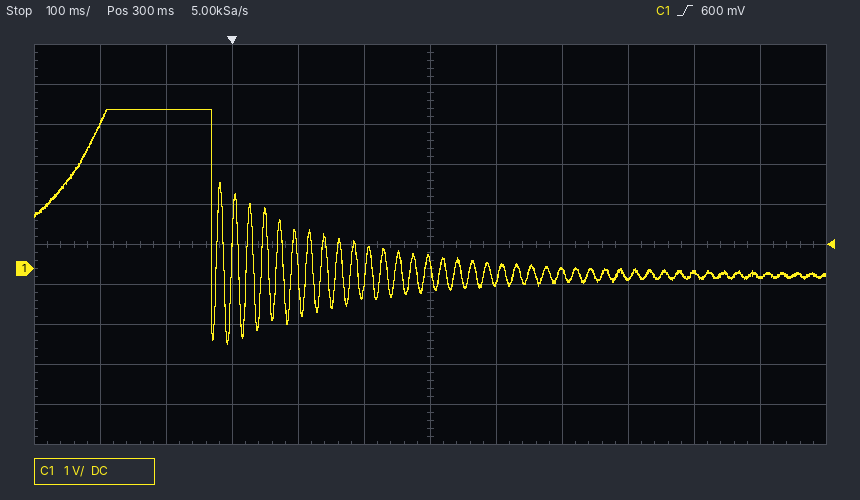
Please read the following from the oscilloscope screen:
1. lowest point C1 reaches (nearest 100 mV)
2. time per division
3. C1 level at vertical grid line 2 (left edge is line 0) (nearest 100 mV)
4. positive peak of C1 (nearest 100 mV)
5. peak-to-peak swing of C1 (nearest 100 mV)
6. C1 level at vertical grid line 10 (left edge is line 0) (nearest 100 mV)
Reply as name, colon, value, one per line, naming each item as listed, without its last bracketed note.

lowest point C1 reaches: -1.9 V
time per division: 100 ms
C1 level at vertical grid line 2 (left edge is line 0): 4.0 V
positive peak of C1: 4.0 V
peak-to-peak swing of C1: 5.9 V
C1 level at vertical grid line 10 (left edge is line 0): -100 mV
